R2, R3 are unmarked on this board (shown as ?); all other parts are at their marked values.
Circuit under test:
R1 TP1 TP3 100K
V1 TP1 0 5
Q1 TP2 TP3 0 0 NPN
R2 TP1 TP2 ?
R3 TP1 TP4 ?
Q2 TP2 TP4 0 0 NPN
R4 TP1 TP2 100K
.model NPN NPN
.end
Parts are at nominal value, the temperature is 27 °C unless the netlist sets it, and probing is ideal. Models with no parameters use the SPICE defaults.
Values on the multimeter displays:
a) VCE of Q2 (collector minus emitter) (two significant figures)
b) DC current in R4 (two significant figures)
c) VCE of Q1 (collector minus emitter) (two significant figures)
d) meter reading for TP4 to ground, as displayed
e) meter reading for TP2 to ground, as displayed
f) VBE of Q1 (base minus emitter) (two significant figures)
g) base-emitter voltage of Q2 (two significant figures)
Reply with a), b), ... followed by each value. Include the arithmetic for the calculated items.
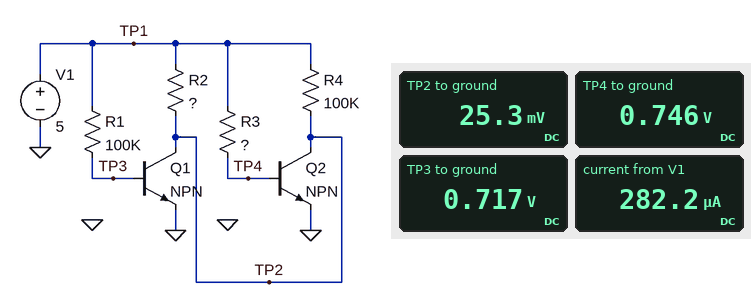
a) 25.3 mV = 25 mV
b) (5 V - 25.3 mV) / 100 kΩ = 50 µA
c) 25.3 mV = 25 mV
d) 0.746 V
e) 25.3 mV
f) 717 mV = 720 mV
g) 746 mV = 750 mV
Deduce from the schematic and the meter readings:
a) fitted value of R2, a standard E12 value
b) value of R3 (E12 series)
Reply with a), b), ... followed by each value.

a) 82 kΩ
b) 33 kΩ
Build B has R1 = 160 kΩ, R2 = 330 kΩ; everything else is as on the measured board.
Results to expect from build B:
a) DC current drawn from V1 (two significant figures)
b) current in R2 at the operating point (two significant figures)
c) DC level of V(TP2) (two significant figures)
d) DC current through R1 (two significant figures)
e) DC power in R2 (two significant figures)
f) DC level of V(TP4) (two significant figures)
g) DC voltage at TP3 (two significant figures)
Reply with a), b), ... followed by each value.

a) 220 µA
b) 15 µA
c) 23 mV
d) 27 µA
e) 75 µW
f) 740 mV
g) 700 mV
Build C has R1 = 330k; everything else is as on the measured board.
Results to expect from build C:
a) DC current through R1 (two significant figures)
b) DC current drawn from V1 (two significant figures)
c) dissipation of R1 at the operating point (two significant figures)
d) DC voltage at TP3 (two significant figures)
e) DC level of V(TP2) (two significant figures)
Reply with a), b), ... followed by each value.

a) 13 µA
b) 250 µA
c) 56 µW
d) 690 mV
e) 27 mV
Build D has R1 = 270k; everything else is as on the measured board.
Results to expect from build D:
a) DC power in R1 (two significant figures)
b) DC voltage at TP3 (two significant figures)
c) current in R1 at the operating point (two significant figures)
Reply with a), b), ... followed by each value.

a) 69 µW
b) 690 mV
c) 16 µA
